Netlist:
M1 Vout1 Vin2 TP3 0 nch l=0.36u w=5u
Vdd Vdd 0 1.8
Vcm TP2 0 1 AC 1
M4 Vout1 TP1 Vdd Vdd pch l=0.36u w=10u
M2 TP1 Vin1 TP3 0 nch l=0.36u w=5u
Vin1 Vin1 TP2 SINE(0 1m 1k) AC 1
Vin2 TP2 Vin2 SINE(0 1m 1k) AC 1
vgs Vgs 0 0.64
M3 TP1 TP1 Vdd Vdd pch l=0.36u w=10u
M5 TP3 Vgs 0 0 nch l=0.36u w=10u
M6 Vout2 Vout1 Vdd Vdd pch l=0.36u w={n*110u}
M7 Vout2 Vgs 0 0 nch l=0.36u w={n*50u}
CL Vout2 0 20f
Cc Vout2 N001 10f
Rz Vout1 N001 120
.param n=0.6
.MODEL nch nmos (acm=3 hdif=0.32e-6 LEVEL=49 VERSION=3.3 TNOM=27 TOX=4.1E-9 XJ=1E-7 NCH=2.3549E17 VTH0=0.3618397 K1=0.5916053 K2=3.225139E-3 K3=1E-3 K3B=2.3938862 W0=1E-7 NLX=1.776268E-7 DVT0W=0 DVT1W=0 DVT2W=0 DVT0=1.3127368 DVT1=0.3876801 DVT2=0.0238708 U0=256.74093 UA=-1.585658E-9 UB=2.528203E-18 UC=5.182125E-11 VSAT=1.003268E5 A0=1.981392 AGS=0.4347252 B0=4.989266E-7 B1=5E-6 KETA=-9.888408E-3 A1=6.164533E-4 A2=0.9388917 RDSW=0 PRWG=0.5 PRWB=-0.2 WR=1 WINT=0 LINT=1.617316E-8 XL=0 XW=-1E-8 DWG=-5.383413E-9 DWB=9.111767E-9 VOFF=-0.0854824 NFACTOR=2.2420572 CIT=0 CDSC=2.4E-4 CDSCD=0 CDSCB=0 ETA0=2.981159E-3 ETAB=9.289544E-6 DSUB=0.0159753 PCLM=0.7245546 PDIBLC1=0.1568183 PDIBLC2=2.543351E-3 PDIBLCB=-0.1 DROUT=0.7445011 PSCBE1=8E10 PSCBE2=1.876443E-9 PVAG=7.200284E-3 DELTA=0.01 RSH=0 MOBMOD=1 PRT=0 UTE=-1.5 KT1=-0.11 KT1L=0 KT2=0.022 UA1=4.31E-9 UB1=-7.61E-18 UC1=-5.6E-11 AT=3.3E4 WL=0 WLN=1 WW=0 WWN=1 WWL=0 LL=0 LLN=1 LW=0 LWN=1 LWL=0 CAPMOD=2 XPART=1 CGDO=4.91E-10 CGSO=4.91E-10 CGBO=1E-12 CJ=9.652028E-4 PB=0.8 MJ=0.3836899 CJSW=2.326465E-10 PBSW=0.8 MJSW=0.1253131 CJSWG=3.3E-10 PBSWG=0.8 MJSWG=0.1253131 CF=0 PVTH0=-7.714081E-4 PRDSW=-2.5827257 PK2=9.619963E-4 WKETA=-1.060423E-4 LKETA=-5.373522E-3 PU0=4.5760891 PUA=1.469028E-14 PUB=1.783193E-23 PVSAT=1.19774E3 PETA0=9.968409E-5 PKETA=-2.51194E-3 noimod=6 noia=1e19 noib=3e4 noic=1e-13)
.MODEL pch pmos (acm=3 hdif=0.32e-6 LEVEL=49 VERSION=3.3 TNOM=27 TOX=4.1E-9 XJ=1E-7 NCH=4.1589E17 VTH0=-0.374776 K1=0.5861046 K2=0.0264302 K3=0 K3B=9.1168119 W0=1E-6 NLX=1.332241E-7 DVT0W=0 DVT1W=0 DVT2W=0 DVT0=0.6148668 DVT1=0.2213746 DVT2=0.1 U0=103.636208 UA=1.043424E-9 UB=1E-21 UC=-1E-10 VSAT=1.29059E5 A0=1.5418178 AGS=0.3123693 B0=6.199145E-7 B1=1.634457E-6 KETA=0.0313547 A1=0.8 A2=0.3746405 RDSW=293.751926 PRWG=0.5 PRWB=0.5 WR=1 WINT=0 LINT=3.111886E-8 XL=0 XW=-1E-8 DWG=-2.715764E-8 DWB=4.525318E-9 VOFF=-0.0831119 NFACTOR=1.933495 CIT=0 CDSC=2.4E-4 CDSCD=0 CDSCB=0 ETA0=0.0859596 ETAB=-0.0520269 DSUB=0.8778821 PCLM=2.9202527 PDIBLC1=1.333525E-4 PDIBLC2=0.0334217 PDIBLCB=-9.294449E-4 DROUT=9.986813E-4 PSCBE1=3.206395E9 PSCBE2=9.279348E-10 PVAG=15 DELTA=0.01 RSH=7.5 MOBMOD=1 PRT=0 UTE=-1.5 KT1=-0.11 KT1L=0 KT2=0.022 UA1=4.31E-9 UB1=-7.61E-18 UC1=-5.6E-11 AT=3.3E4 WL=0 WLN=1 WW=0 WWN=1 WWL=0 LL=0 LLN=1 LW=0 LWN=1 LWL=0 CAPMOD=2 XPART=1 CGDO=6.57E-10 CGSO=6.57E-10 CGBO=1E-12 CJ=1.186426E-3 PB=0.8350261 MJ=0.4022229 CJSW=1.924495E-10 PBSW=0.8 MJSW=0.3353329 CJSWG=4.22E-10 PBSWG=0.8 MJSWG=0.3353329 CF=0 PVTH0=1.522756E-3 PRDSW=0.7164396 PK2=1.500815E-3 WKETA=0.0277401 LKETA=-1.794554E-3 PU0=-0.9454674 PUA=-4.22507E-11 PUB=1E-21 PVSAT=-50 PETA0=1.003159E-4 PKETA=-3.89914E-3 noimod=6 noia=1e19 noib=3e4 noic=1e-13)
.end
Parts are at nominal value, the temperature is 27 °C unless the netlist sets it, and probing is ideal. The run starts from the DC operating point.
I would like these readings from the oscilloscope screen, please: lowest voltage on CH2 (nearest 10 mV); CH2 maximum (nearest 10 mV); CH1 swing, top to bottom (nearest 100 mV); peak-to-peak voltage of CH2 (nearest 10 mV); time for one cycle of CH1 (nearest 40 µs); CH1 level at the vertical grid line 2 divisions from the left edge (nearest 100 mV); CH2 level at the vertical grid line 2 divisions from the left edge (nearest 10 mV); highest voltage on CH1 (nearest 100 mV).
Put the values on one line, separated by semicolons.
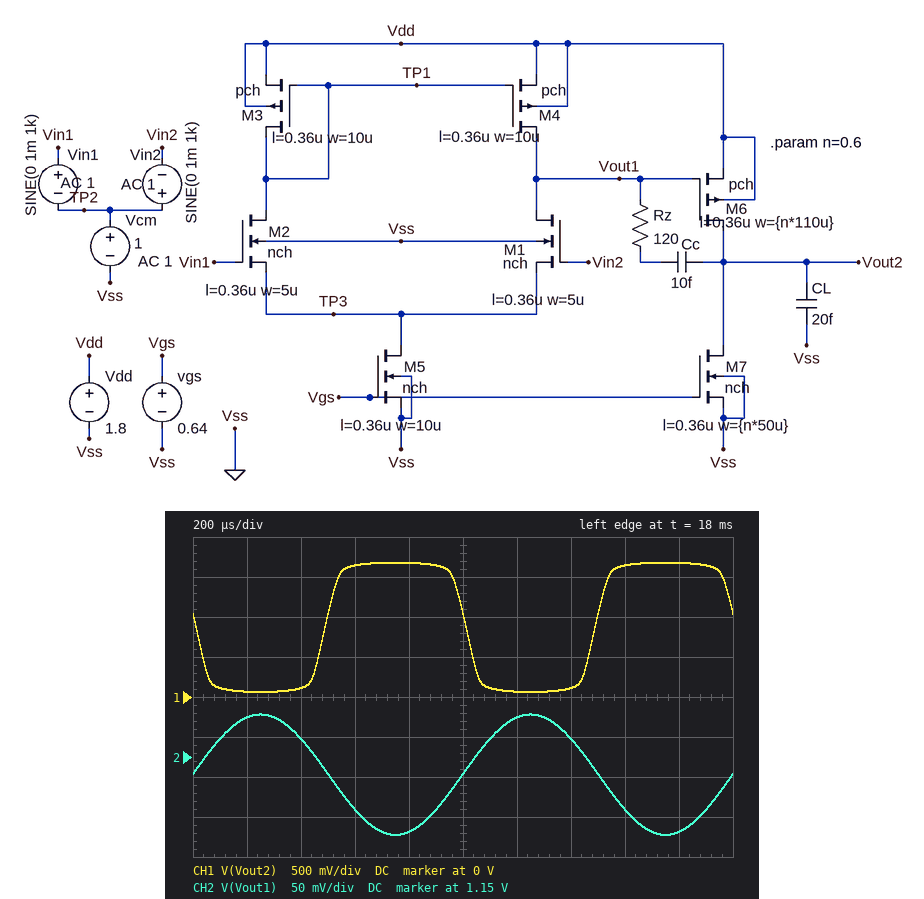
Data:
1.05 V; 1.20 V; 1.6 V; 150 mV; 1.00 ms; 100 mV; 1.17 V; 1.7 V
